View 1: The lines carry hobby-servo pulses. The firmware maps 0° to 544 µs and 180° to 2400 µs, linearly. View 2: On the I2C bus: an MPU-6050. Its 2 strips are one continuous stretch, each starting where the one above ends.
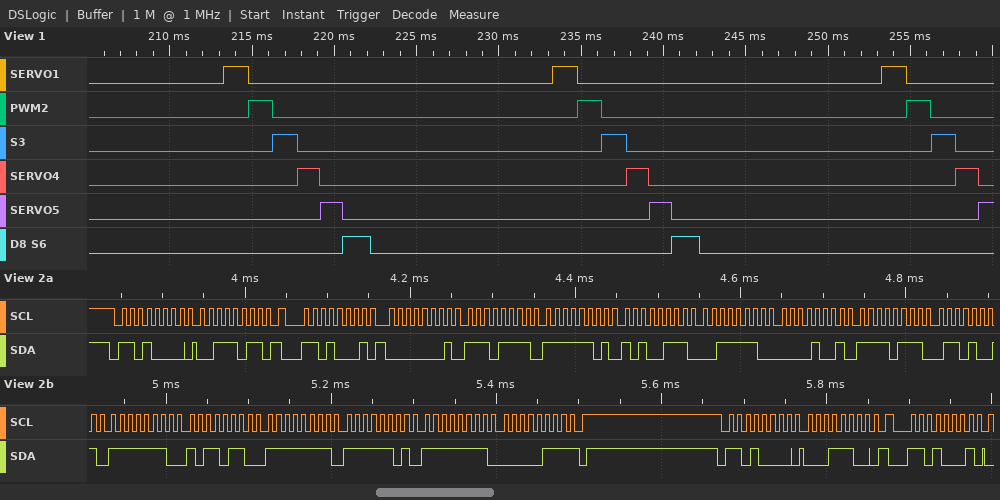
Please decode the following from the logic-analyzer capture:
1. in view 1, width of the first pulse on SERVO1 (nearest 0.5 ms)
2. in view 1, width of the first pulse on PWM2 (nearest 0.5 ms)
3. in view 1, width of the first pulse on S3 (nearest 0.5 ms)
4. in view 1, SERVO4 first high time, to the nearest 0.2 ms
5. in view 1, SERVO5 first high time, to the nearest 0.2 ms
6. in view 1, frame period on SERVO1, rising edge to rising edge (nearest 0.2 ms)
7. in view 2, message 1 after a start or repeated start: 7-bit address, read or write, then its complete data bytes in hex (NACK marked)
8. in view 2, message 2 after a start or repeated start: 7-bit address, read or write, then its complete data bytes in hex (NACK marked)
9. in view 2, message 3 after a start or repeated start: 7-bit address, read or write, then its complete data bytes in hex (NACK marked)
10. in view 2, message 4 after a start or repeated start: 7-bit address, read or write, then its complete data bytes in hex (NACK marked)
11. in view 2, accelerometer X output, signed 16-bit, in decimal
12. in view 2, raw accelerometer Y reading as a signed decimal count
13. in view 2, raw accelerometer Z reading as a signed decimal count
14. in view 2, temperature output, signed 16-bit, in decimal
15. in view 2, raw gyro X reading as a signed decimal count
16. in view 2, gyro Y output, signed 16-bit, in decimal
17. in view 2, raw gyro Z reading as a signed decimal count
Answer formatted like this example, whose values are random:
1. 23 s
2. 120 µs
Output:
1. 1.5 ms
2. 1.5 ms
3. 1.5 ms
4. 1.4 ms
5. 1.4 ms
6. 20.0 ms
7. 0x68 write: 3B
8. 0x68 read: 01 EF FD A7 3E 09 F7 69 FE B6 FF FD FF 07 NACK
9. 0x68 write: 1C
10. 0x68 read
11. 495
12. -601
13. 15881
14. -2199
15. -330
16. -3
17. -249
